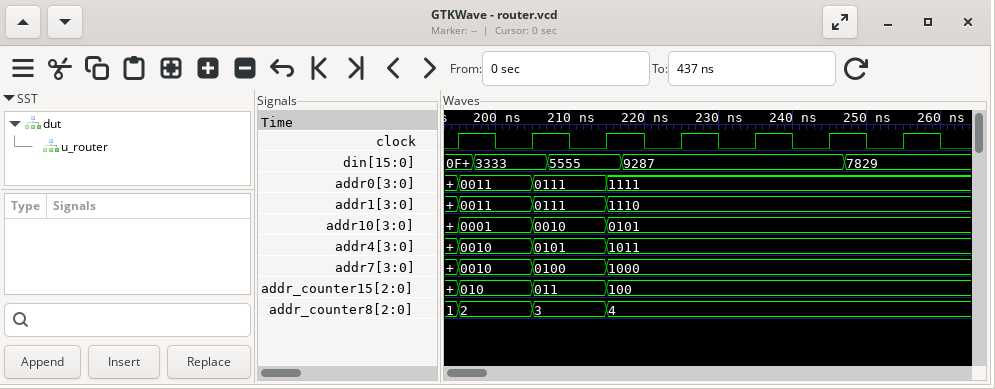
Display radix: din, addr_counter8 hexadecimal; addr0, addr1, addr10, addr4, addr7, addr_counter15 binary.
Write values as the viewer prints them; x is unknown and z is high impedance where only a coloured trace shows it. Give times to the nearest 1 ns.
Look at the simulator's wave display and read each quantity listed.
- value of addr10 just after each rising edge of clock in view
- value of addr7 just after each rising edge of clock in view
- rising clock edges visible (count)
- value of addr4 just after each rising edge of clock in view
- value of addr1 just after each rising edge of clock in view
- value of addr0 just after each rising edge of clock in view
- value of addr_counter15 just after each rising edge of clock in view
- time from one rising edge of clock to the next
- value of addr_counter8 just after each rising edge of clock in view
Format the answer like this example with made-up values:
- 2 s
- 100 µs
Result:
- 0001, 0010, 0101, 0101, 0101, 0101, 0101
- 0010, 0100, 1000, 1000, 1000, 1000, 1000
- 7
- 0010, 0101, 1011, 1011, 1011, 1011, 1011
- 0011, 0111, 1110, 1110, 1110, 1110, 1110
- 0011, 0111, 1111, 1111, 1111, 1111, 1111
- 010, 011, 100, 100, 100, 100, 100
- 10 ns
- 2, 3, 4, 4, 4, 4, 4
